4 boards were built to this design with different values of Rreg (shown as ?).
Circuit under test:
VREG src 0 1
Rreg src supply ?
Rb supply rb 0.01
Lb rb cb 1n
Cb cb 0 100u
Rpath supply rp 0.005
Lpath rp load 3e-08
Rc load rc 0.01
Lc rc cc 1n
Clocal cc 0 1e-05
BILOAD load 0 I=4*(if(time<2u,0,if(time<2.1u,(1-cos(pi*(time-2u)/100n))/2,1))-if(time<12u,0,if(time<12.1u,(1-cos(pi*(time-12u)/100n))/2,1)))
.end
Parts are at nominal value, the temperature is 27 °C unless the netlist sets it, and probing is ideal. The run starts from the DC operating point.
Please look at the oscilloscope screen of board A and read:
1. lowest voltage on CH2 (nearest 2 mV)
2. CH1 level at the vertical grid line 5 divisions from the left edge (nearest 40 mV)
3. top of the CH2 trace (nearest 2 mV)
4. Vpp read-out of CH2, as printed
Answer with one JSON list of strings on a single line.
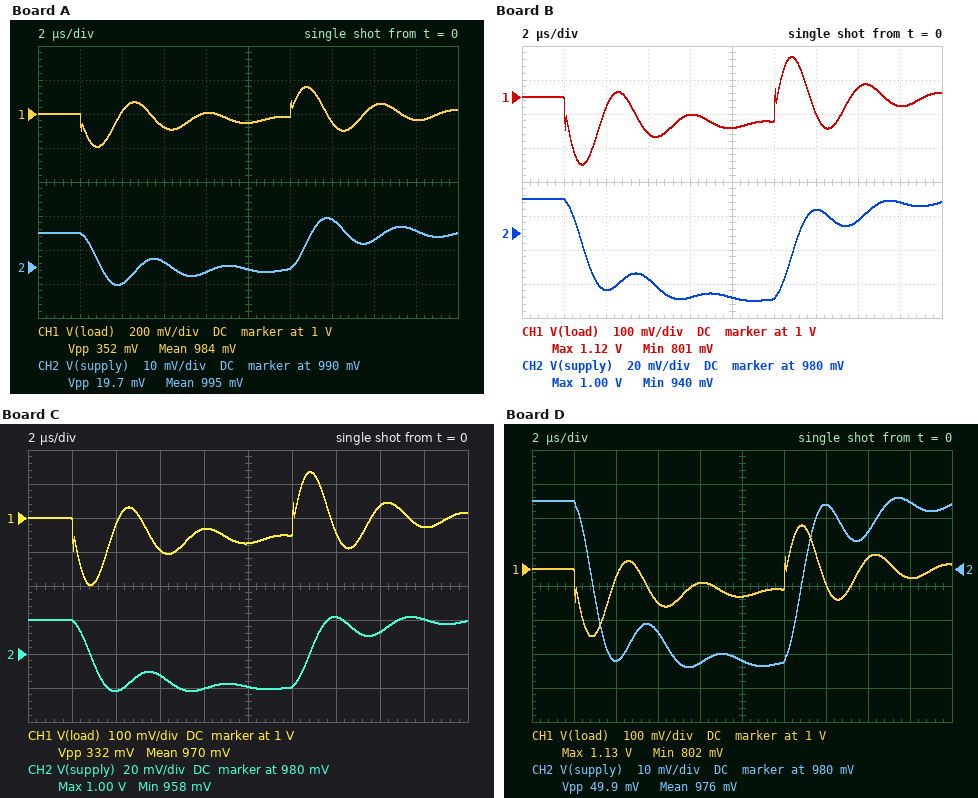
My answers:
["984 mV", "960 mV", "1.004 V", "19.7 mV"]
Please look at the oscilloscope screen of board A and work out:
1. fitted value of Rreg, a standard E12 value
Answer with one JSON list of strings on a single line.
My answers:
["2.7 mΩ"]
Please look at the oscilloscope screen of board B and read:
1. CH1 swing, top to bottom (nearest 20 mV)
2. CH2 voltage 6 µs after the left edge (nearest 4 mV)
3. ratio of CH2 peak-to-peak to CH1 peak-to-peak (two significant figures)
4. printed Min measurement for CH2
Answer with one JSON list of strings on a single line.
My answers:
["320 mV", "952 mV", "0.19", "940 mV"]
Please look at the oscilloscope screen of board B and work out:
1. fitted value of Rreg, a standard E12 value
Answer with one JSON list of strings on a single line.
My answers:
["0.015 Ω"]
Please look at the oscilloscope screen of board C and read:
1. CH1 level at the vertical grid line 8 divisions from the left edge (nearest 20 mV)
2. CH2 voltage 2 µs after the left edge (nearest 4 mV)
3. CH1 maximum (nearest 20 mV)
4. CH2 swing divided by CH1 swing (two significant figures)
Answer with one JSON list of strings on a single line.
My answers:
["1.04 V", "1.000 V", "1.14 V", "0.13"]
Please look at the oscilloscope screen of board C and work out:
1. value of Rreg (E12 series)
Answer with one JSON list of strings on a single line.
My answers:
["0.01 Ω"]
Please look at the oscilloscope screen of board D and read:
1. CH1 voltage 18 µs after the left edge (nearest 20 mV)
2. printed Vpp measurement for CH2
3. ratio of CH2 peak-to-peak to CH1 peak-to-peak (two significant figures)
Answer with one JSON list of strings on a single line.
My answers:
["980 mV", "49.9 mV", "0.15"]
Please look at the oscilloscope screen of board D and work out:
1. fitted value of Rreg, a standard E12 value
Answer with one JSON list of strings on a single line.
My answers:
["0.012 Ω"]
